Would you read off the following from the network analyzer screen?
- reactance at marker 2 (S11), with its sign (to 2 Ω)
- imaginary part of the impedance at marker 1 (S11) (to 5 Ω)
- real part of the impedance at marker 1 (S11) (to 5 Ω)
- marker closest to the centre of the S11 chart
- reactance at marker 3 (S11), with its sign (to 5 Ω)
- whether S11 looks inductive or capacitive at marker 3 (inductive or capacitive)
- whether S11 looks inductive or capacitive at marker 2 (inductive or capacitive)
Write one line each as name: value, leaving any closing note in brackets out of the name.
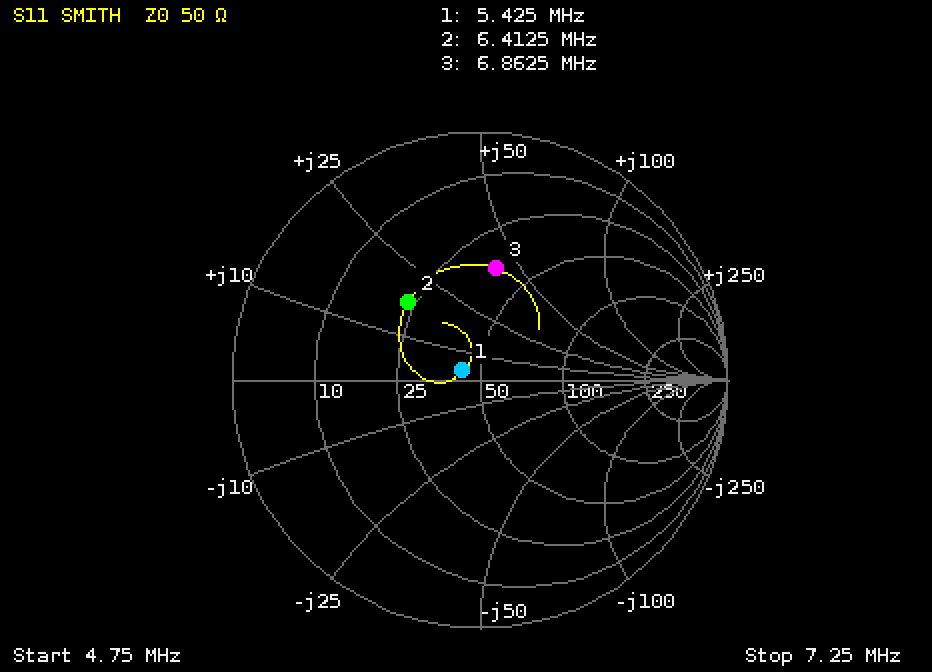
reactance at marker 2 (S11), with its sign: +18 Ω
imaginary part of the impedance at marker 1 (S11): +5 Ω
real part of the impedance at marker 1 (S11): 45 Ω
marker closest to the centre of the S11 chart: marker 1
reactance at marker 3 (S11), with its sign: +40 Ω
whether S11 looks inductive or capacitive at marker 3: inductive
whether S11 looks inductive or capacitive at marker 2: inductive
